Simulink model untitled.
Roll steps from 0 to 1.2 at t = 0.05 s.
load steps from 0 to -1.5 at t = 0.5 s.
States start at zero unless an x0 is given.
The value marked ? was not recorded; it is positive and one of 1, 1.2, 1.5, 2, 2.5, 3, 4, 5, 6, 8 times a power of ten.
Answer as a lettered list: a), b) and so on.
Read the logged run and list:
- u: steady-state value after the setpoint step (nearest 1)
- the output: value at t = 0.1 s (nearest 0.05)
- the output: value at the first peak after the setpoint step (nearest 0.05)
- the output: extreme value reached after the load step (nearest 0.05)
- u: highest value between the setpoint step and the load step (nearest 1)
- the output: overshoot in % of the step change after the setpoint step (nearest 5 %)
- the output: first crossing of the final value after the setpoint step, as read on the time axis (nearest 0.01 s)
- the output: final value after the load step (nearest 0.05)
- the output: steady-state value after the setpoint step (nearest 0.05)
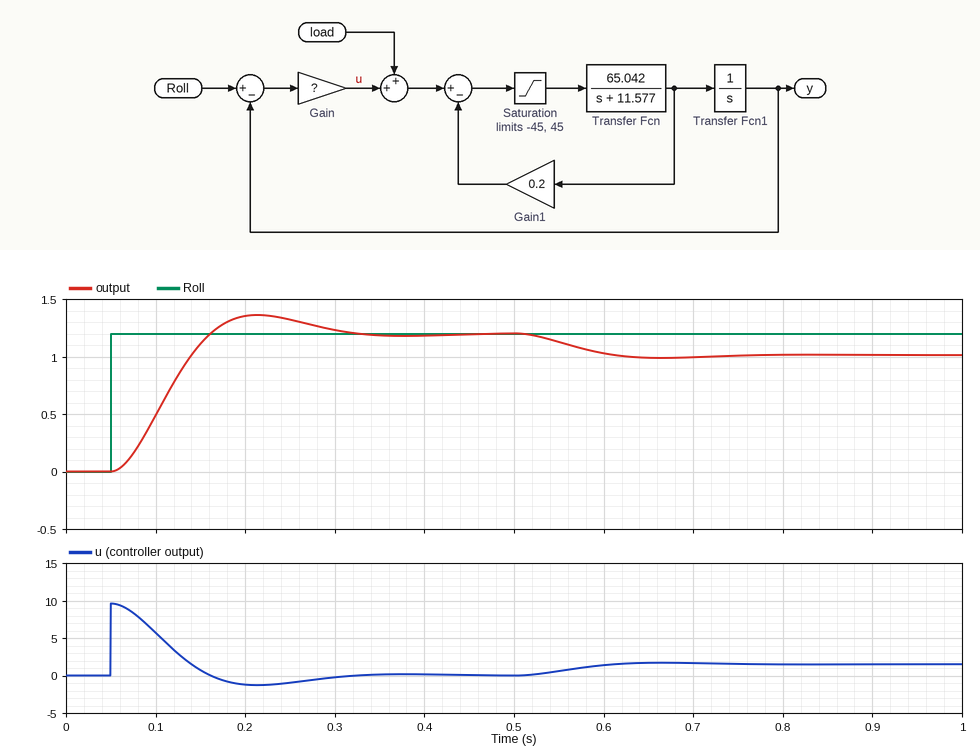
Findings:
a) 0
b) 0.50
c) 1.35
d) 1.00
e) 10
f) 15 %
g) 0.16 s
h) 1.00
i) 1.20
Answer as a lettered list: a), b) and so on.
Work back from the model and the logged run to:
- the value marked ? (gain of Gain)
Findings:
a) 8
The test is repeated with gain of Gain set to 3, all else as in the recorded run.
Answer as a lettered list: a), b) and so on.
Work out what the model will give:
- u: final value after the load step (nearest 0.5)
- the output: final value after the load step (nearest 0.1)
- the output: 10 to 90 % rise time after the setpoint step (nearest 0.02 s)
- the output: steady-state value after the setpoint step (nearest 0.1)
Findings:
a) 1.5
b) 0.7
c) 0.20 s
d) 1.2
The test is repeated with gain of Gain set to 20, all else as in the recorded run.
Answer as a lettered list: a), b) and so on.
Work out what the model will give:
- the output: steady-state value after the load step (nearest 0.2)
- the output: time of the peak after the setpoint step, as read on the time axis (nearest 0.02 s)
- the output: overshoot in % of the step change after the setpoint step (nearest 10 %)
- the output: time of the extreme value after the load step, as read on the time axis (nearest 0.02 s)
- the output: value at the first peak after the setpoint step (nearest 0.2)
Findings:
a) 1.2
b) 0.14 s
c) 30 %
d) 0.60 s
e) 1.6
